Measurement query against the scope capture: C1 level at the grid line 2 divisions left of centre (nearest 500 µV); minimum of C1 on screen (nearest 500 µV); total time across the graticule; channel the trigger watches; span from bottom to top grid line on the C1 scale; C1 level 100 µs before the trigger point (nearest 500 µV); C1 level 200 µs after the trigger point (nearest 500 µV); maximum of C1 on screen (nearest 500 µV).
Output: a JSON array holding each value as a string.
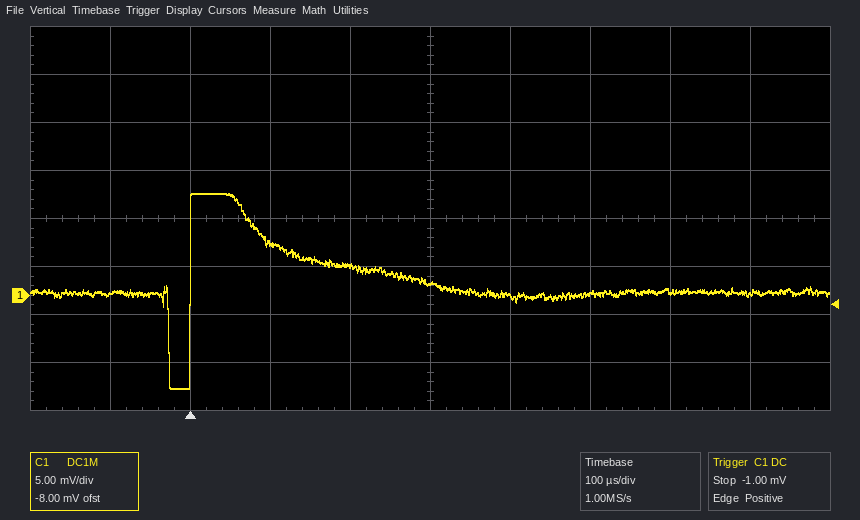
["5.5 mV", "-9.5 mV", "1 ms", "C1", "40 mV", "0.0 mV", "3.0 mV", "10.5 mV"]
